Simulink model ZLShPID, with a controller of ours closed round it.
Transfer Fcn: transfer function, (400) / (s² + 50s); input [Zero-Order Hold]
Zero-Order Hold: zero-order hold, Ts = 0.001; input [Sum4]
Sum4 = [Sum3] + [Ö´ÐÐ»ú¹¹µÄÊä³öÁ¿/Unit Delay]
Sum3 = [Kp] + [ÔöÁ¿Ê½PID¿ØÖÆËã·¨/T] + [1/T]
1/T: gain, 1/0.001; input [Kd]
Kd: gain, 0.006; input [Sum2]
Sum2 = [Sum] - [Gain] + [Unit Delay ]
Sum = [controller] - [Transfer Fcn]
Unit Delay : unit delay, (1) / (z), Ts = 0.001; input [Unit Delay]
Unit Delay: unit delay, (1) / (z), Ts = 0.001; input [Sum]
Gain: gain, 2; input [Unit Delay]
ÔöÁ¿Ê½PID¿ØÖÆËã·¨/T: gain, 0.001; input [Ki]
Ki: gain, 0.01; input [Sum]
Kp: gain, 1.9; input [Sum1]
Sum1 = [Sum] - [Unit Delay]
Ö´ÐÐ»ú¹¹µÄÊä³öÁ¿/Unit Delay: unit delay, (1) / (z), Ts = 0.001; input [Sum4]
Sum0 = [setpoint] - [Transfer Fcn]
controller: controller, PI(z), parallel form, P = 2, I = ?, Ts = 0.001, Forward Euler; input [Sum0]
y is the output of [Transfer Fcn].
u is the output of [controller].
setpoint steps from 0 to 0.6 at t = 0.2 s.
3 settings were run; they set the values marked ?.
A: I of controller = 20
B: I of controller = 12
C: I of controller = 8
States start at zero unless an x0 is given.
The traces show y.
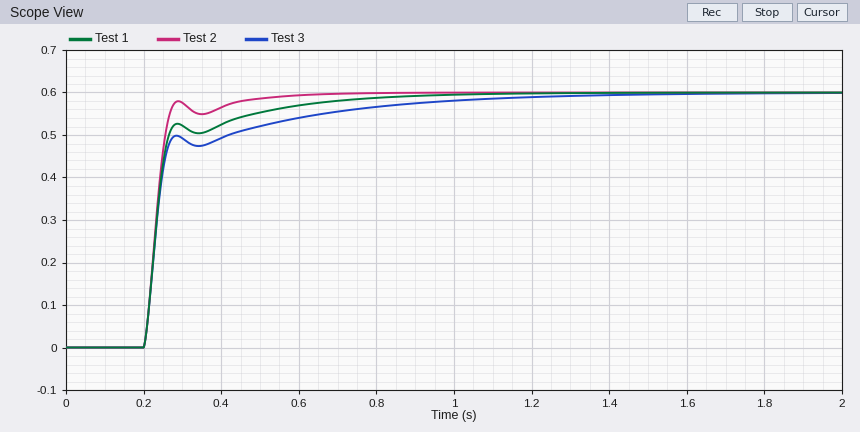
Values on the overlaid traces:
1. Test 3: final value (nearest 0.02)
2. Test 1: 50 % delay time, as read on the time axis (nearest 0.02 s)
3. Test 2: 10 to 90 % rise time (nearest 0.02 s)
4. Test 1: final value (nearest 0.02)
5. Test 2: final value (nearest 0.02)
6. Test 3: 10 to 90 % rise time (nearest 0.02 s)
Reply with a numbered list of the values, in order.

1. 0.60
2. 0.24 s
3. 0.06 s
4. 0.60
5. 0.60
6. 0.38 s
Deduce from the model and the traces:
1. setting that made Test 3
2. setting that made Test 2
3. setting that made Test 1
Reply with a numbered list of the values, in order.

1. C
2. A
3. B
